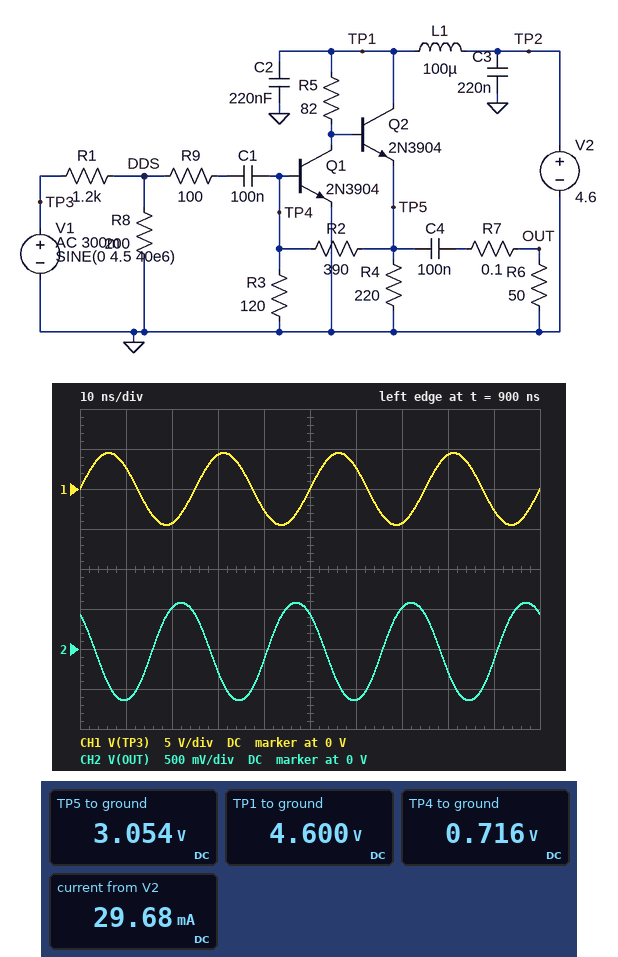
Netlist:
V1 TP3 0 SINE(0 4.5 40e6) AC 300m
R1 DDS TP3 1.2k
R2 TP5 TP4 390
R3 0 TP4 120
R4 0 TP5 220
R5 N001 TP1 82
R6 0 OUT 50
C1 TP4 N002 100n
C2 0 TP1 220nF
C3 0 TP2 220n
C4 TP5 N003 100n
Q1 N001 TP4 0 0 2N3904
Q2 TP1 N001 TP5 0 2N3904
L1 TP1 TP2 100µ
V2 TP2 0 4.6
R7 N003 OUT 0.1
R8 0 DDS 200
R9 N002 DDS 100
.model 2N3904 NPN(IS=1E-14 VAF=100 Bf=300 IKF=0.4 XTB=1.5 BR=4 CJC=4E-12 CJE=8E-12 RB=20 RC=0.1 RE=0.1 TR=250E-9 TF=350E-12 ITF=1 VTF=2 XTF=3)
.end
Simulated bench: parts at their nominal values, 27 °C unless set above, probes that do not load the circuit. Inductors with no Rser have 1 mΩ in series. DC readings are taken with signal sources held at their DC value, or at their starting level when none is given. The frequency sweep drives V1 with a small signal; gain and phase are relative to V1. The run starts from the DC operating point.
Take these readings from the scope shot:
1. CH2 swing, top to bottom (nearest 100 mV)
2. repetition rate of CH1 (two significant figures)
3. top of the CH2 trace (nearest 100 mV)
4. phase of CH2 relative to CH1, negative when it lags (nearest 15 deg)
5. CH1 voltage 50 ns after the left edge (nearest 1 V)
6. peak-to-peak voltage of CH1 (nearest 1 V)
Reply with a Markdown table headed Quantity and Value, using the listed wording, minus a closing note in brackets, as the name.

| Quantity | Value |
|---|---|
| CH2 swing, top to bottom | 1.2 V |
| repetition rate of CH1 | 40 MHz |
| top of the CH2 trace | 600 mV |
| phase of CH2 relative to CH1, negative when it lags | 135 deg |
| CH1 voltage 50 ns after the left edge | 0 V |
| peak-to-peak voltage of CH1 | 9 V |
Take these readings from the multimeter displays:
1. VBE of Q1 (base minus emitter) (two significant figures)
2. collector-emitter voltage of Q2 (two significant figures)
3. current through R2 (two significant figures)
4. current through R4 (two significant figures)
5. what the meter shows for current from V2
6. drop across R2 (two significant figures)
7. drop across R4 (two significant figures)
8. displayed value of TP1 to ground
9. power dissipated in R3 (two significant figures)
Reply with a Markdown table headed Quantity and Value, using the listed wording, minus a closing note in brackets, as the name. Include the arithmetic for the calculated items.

| Quantity | Value |
|---|---|
| VBE of Q1 (base minus emitter) | 716 mV = 720 mV |
| collector-emitter voltage of Q2 | 4.6 V - 3.054 V = 1.5 V |
| current through R2 | (3.054 V - 716 mV) / 390 Ω = 6.0 mA |
| current through R4 | (3.054 V) / 220 Ω = 14 mA |
| what the meter shows for current from V2 | 29.68 mA |
| drop across R2 | 3.054 V - 716 mV = 2.3 V |
| drop across R4 | 3.054 V = 3.1 V |
| displayed value of TP1 to ground | 4.600 V |
| power dissipated in R3 | (716 mV)^2 / 120 Ω = 4.3 mW |
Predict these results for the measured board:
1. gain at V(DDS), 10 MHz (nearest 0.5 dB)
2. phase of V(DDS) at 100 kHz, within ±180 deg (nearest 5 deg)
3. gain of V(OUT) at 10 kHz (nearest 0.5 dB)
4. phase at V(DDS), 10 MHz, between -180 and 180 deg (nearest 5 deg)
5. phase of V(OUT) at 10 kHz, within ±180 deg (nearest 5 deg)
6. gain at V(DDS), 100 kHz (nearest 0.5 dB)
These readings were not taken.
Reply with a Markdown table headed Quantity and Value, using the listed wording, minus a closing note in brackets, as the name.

| Quantity | Value |
|---|---|
| gain at V(DDS), 10 MHz | -25.0 dB |
| phase of V(DDS) at 100 kHz, within ±180 deg | -5 deg |
| gain of V(OUT) at 10 kHz | -27.0 dB |
| phase at V(DDS), 10 MHz, between -180 and 180 deg | 0 deg |
| phase of V(OUT) at 10 kHz, within ±180 deg | -80 deg |
| gain at V(DDS), 100 kHz | -25.0 dB |
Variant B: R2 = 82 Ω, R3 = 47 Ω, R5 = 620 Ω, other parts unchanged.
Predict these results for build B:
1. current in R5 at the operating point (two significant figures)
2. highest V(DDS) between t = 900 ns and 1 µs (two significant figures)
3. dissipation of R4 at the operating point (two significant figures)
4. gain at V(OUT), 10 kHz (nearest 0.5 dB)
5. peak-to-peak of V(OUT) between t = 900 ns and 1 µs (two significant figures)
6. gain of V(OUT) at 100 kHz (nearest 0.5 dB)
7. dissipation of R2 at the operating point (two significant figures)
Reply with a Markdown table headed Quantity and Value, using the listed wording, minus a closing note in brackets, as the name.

| Quantity | Value |
|---|---|
| current in R5 at the operating point | 3.2 mA |
| highest V(DDS) between t = 900 ns and 1 µs | 240 mV |
| dissipation of R4 at the operating point | 16 mW |
| gain at V(OUT), 10 kHz | -39.5 dB |
| peak-to-peak of V(OUT) between t = 900 ns and 1 µs | 390 mV |
| gain of V(OUT) at 100 kHz | -28.0 dB |
| dissipation of R2 at the operating point | 17 mW |
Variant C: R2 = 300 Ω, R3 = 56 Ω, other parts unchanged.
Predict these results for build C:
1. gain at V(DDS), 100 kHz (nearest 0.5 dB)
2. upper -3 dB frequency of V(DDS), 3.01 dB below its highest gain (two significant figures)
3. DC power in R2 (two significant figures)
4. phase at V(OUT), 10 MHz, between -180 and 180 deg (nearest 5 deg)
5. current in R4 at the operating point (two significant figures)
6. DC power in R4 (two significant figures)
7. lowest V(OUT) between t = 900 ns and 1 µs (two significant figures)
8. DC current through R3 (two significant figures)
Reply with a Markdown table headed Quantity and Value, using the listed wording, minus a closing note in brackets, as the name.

| Quantity | Value |
|---|---|
| gain at V(DDS), 100 kHz | -23.5 dB |
| upper -3 dB frequency of V(DDS), 3.01 dB below its highest gain | 6.6 kHz |
| DC power in R2 | 35 mW |
| phase at V(OUT), 10 MHz, between -180 and 180 deg | 170 deg |
| current in R4 at the operating point | 17 mA |
| DC power in R4 | 67 mW |
| lowest V(OUT) between t = 900 ns and 1 µs | -130 mV |
| DC current through R3 | 11 mA |
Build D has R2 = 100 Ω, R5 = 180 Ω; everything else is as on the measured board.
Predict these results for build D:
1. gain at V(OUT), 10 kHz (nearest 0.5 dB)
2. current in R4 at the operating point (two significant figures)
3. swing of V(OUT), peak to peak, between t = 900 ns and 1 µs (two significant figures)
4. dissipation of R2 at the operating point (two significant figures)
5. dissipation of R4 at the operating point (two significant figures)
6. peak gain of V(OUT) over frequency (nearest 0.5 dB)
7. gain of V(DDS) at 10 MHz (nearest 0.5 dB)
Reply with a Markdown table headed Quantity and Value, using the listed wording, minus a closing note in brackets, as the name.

| Quantity | Value |
|---|---|
| gain at V(OUT), 10 kHz | -37.5 dB |
| current in R4 at the operating point | 6.1 mA |
| swing of V(OUT), peak to peak, between t = 900 ns and 1 µs | 480 mV |
| dissipation of R2 at the operating point | 3.7 mW |
| dissipation of R4 at the operating point | 8.1 mW |
| peak gain of V(OUT) over frequency | -24.0 dB |
| gain of V(DDS) at 10 MHz | -25.5 dB |
